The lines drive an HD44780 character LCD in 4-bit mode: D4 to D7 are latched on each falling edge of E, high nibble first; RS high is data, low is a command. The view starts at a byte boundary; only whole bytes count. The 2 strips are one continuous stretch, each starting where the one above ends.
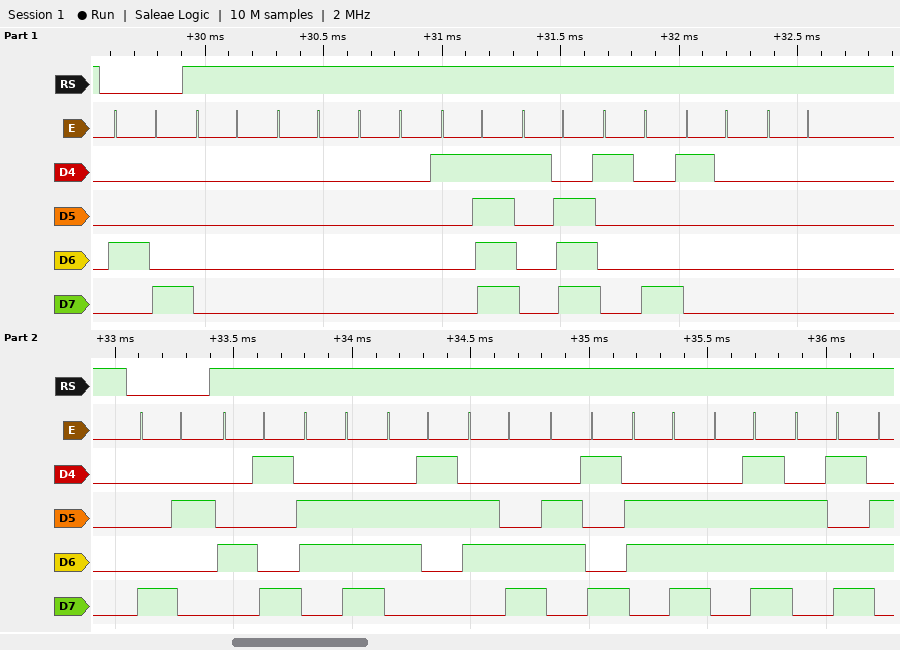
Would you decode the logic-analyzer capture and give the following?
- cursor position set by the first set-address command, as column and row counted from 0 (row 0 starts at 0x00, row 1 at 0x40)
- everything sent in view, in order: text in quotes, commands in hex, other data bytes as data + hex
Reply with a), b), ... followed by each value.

a) column 2, row 0
b) 0x48 data 00 00 00 1F 1E 18 10 00 0x82 "Inclinom"
